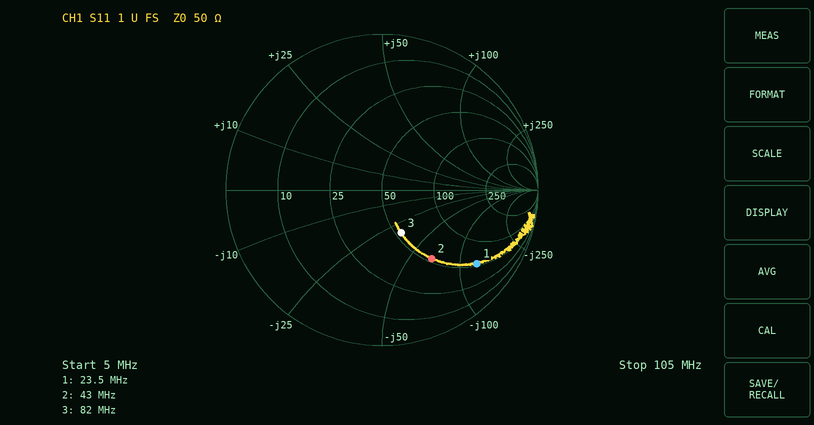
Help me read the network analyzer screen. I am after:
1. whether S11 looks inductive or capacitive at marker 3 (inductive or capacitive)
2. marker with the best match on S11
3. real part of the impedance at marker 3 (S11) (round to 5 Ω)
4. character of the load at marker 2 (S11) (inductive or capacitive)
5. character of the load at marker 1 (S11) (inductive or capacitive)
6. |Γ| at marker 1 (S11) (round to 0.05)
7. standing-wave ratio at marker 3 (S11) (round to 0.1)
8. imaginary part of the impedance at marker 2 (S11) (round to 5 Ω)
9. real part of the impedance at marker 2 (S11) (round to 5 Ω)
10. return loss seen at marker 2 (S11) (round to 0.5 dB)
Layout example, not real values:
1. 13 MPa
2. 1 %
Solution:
1. capacitive
2. marker 3
3. 55 Ω
4. capacitive
5. capacitive
6. 0.75
7. 1.9
8. -65 Ω
9. 55 Ω
10. 5.5 dB
